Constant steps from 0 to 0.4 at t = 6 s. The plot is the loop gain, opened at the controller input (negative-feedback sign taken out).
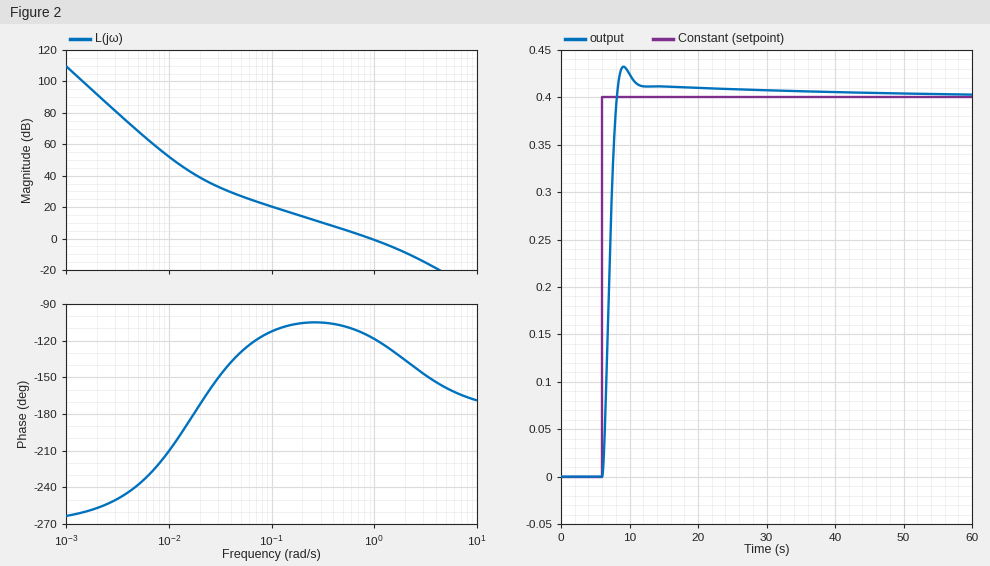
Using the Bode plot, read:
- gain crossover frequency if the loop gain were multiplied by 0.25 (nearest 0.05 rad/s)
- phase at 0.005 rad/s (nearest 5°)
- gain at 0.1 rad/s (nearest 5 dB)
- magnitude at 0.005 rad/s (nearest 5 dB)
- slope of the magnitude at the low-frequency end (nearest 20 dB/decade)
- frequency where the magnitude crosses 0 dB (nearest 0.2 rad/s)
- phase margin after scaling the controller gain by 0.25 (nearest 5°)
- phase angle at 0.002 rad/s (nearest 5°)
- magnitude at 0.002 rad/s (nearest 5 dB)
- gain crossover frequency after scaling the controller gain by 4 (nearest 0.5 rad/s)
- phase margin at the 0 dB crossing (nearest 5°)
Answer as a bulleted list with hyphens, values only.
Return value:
- 0.25 rad/s
- -240°
- 20 dB
- 70 dB
- -60 dB/decade
- 1.0 rad/s
- 75°
- -255°
- 90 dB
- 2.5 rad/s
- 65°
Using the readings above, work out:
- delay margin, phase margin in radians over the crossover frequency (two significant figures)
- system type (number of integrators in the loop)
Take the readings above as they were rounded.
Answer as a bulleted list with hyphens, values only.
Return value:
- 1.1 s
- 3
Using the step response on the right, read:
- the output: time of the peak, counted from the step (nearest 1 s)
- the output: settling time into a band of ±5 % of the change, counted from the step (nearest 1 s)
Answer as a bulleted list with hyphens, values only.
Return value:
- 3 s
- 4 s
